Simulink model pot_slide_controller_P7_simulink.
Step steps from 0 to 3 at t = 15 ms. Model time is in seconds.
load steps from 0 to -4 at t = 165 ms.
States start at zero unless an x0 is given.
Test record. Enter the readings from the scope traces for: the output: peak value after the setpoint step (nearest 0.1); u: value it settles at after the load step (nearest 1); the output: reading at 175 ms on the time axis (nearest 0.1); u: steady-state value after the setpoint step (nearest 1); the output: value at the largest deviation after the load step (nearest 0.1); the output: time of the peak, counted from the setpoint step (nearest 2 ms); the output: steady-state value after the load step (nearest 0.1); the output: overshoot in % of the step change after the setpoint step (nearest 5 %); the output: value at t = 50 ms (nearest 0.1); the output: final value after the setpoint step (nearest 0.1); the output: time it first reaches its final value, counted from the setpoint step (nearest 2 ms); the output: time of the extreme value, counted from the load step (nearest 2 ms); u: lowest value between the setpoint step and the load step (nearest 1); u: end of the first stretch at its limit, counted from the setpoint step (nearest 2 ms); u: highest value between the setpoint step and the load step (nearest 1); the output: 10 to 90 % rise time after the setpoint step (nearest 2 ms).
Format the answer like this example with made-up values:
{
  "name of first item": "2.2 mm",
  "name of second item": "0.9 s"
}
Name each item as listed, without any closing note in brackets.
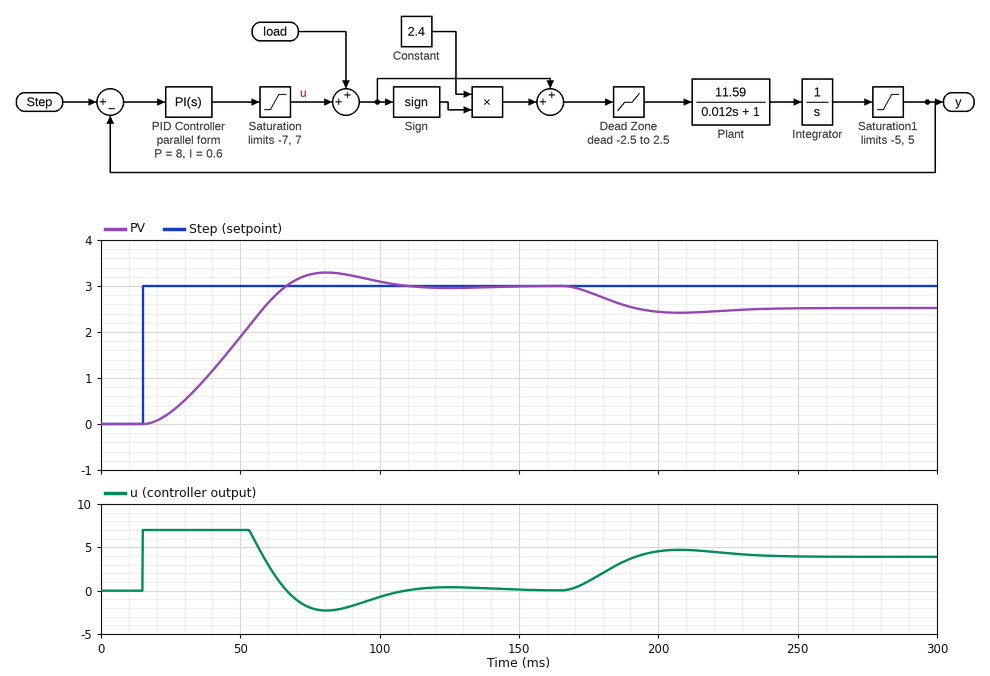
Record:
{
  "the output: peak value after the setpoint step": "3.3",
  "u: value it settles at after the load step": "4",
  "the output: reading at 175 ms on the time axis": "2.9",
  "u: steady-state value after the setpoint step": "0",
  "the output: value at the largest deviation after the load step": "2.4",
  "the output: time of the peak, counted from the setpoint step": "66 ms",
  "the output: steady-state value after the load step": "2.5",
  "the output: overshoot in % of the step change after the setpoint step": "10 %",
  "the output: value at t = 50 ms": "1.9",
  "the output: final value after the setpoint step": "3.0",
  "the output: time it first reaches its final value, counted from the setpoint step": "52 ms",
  "the output: time of the extreme value, counted from the load step": "42 ms",
  "u: lowest value between the setpoint step and the load step": "-2",
  "u: end of the first stretch at its limit, counted from the setpoint step": "38 ms",
  "u: highest value between the setpoint step and the load step": "7",
  "the output: 10 to 90 % rise time after the setpoint step": "36 ms"
}
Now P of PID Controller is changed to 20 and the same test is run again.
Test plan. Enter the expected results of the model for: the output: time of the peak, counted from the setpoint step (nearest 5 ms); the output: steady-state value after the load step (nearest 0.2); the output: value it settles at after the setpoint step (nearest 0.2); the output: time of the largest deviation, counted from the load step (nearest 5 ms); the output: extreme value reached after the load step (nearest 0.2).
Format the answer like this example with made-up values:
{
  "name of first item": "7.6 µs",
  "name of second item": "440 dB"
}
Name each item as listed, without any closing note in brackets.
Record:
{
  "the output: time of the peak, counted from the setpoint step": "60 ms",
  "the output: steady-state value after the load step": "2.8",
  "the output: value it settles at after the setpoint step": "3.0",
  "the output: time of the largest deviation, counted from the load step": "25 ms",
  "the output: extreme value reached after the load step": "2.8"
}
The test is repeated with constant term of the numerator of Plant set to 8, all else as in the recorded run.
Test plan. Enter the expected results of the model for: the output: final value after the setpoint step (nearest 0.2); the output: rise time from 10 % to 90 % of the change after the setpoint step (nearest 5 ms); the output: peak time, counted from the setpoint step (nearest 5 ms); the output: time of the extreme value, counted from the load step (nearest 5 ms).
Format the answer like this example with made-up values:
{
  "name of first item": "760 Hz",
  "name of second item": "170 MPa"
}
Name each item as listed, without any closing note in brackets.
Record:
{
  "the output: final value after the setpoint step": "3.0",
  "the output: rise time from 10 % to 90 % of the change after the setpoint step": "50 ms",
  "the output: peak time, counted from the setpoint step": "90 ms",
  "the output: time of the extreme value, counted from the load step": "55 ms"
}
